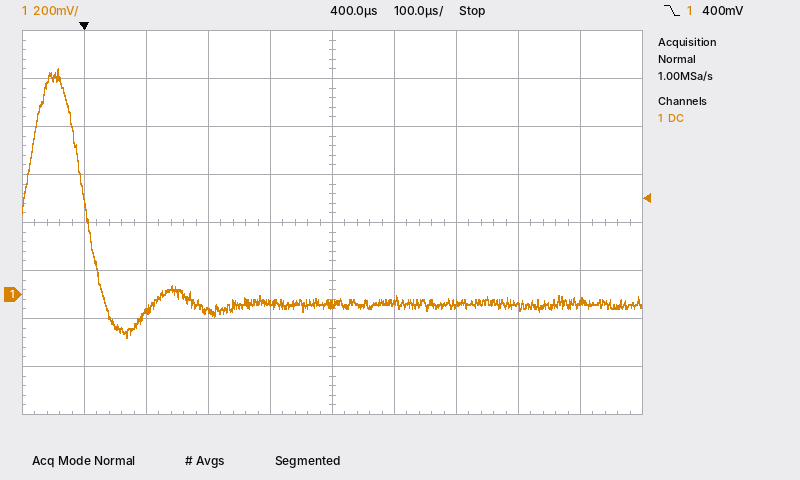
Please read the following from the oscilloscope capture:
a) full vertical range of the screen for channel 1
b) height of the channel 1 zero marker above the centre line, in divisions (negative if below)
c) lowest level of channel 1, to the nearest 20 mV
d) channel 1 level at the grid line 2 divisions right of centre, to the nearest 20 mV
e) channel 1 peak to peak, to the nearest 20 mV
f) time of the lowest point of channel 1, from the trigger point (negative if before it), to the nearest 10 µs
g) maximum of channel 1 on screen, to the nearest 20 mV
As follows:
1.6 V
-1.5 div
-180 mV
-40 mV
1.12 V
+70 µs
940 mV
